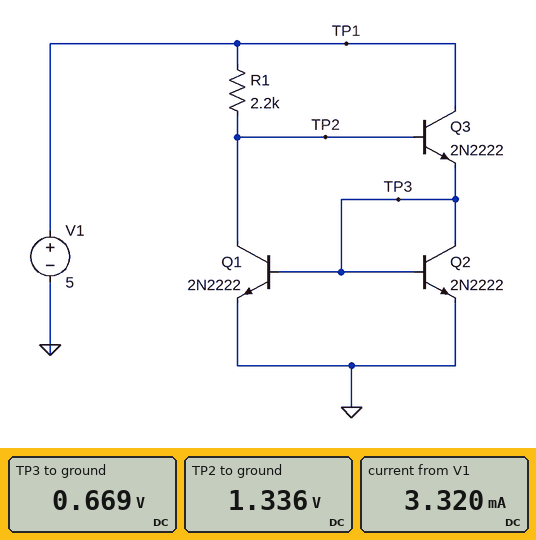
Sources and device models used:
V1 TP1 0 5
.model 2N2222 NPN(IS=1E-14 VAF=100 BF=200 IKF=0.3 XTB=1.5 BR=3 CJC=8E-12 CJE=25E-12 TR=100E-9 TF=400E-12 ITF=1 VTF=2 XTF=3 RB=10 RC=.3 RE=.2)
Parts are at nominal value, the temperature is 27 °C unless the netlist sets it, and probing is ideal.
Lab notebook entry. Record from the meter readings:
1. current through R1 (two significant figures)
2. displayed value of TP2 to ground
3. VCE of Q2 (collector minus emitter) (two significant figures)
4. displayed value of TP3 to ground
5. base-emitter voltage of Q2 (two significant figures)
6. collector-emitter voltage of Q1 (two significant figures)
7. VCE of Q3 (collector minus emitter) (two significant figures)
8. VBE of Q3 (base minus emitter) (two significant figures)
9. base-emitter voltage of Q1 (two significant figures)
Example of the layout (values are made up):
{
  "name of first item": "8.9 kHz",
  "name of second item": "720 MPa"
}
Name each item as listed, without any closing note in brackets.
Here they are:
{
  "current through R1": "1.7 mA",
  "displayed value of TP2 to ground": "1.336 V",
  "VCE of Q2 (collector minus emitter)": "670 mV",
  "displayed value of TP3 to ground": "0.669 V",
  "base-emitter voltage of Q2": "670 mV",
  "collector-emitter voltage of Q1": "1.3 V",
  "VCE of Q3 (collector minus emitter)": "4.3 V",
  "VBE of Q3 (base minus emitter)": "670 mV",
  "base-emitter voltage of Q1": "670 mV"
}
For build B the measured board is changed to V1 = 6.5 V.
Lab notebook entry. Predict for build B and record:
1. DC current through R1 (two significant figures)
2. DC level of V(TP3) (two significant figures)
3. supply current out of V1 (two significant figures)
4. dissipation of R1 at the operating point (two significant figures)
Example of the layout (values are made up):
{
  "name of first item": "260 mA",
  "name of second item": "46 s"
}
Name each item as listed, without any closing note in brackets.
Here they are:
{
  "DC current through R1": "2.3 mA",
  "DC level of V(TP3)": "680 mV",
  "supply current out of V1": "4.7 mA",
  "dissipation of R1 at the operating point": "12 mW"
}
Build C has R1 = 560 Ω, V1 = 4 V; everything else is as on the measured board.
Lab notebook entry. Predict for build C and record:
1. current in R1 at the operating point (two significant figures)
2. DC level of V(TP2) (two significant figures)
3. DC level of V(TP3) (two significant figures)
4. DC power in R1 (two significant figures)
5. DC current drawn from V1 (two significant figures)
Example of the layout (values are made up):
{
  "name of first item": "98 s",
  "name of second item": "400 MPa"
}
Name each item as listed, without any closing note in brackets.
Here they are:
{
  "current in R1 at the operating point": "4.7 mA",
  "DC level of V(TP2)": "1.4 V",
  "DC level of V(TP3)": "700 mV",
  "DC power in R1": "12 mW",
  "DC current drawn from V1": "9.3 mA"
}
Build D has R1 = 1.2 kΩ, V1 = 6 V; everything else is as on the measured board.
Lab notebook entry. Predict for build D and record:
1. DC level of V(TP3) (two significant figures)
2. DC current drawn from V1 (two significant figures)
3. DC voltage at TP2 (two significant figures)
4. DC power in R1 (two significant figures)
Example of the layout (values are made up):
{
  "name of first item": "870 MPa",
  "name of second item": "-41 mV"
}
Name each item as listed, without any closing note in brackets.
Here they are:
{
  "DC level of V(TP3)": "690 mV",
  "DC current drawn from V1": "7.7 mA",
  "DC voltage at TP2": "1.4 V",
  "DC power in R1": "18 mW"
}
